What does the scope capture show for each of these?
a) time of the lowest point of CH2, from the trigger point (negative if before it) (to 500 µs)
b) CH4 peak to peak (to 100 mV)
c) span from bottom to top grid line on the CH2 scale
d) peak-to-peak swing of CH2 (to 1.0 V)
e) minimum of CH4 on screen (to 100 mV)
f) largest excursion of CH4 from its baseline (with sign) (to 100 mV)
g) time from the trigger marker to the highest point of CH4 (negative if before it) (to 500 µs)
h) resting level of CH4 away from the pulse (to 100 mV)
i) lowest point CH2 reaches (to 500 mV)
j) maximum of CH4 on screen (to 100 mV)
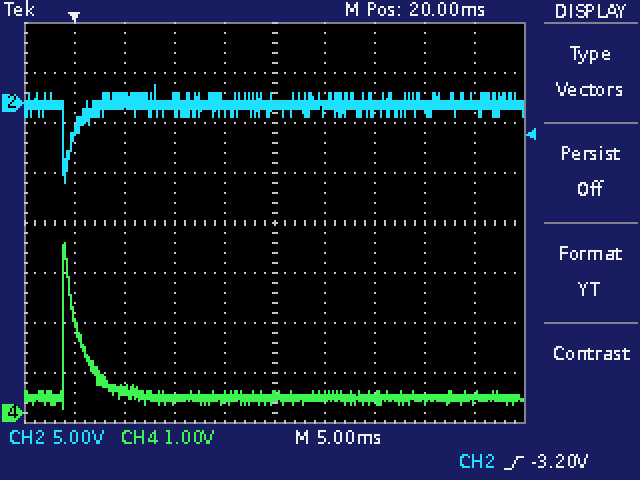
-1.0 ms
3.3 V
40 V
10.0 V
100 mV
+3.1 V
-1.0 ms
300 mV
-8.0 V
3.4 V
